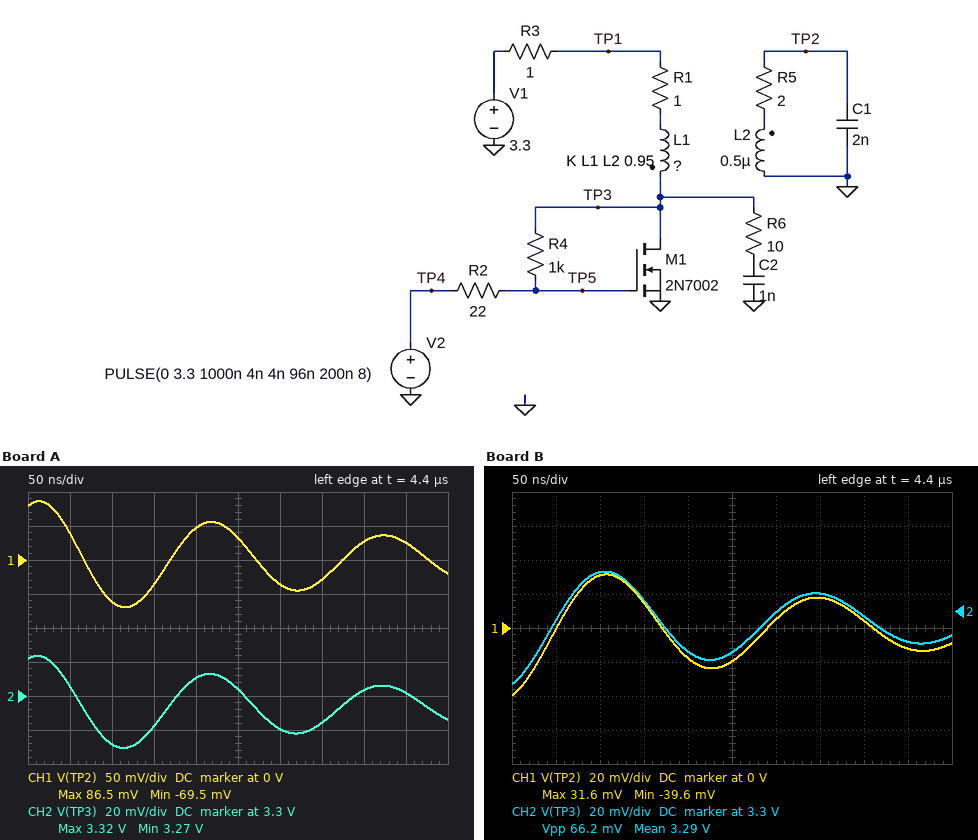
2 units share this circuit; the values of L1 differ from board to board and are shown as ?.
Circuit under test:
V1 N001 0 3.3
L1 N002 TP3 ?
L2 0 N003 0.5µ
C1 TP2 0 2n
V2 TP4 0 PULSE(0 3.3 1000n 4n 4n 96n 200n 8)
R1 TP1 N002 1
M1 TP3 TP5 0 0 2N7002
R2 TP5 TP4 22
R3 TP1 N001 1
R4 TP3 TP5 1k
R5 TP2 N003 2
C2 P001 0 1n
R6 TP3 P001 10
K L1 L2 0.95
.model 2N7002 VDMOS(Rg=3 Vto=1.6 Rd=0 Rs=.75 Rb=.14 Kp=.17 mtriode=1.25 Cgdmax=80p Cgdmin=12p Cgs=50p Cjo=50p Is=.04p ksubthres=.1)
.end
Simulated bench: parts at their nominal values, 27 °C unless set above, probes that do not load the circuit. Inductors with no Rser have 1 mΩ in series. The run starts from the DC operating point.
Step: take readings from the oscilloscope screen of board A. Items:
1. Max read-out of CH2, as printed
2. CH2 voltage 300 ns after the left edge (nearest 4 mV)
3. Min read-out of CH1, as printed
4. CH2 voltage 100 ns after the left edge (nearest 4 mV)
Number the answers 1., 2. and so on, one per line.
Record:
1. 3.32 V
2. 3.280 V
3. -69.5 mV
4. 3.272 V
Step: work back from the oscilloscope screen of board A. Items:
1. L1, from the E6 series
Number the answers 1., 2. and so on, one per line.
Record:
1. 68 nH
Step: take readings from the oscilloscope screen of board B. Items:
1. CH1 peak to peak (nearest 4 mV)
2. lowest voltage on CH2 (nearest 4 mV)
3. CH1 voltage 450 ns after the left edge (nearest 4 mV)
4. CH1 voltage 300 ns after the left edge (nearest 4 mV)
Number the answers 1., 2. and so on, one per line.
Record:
1. 72 mV
2. 3.256 V
3. -12 mV
4. 4 mV
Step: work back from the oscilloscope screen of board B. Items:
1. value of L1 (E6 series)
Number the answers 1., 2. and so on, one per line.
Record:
1. 470 nH
